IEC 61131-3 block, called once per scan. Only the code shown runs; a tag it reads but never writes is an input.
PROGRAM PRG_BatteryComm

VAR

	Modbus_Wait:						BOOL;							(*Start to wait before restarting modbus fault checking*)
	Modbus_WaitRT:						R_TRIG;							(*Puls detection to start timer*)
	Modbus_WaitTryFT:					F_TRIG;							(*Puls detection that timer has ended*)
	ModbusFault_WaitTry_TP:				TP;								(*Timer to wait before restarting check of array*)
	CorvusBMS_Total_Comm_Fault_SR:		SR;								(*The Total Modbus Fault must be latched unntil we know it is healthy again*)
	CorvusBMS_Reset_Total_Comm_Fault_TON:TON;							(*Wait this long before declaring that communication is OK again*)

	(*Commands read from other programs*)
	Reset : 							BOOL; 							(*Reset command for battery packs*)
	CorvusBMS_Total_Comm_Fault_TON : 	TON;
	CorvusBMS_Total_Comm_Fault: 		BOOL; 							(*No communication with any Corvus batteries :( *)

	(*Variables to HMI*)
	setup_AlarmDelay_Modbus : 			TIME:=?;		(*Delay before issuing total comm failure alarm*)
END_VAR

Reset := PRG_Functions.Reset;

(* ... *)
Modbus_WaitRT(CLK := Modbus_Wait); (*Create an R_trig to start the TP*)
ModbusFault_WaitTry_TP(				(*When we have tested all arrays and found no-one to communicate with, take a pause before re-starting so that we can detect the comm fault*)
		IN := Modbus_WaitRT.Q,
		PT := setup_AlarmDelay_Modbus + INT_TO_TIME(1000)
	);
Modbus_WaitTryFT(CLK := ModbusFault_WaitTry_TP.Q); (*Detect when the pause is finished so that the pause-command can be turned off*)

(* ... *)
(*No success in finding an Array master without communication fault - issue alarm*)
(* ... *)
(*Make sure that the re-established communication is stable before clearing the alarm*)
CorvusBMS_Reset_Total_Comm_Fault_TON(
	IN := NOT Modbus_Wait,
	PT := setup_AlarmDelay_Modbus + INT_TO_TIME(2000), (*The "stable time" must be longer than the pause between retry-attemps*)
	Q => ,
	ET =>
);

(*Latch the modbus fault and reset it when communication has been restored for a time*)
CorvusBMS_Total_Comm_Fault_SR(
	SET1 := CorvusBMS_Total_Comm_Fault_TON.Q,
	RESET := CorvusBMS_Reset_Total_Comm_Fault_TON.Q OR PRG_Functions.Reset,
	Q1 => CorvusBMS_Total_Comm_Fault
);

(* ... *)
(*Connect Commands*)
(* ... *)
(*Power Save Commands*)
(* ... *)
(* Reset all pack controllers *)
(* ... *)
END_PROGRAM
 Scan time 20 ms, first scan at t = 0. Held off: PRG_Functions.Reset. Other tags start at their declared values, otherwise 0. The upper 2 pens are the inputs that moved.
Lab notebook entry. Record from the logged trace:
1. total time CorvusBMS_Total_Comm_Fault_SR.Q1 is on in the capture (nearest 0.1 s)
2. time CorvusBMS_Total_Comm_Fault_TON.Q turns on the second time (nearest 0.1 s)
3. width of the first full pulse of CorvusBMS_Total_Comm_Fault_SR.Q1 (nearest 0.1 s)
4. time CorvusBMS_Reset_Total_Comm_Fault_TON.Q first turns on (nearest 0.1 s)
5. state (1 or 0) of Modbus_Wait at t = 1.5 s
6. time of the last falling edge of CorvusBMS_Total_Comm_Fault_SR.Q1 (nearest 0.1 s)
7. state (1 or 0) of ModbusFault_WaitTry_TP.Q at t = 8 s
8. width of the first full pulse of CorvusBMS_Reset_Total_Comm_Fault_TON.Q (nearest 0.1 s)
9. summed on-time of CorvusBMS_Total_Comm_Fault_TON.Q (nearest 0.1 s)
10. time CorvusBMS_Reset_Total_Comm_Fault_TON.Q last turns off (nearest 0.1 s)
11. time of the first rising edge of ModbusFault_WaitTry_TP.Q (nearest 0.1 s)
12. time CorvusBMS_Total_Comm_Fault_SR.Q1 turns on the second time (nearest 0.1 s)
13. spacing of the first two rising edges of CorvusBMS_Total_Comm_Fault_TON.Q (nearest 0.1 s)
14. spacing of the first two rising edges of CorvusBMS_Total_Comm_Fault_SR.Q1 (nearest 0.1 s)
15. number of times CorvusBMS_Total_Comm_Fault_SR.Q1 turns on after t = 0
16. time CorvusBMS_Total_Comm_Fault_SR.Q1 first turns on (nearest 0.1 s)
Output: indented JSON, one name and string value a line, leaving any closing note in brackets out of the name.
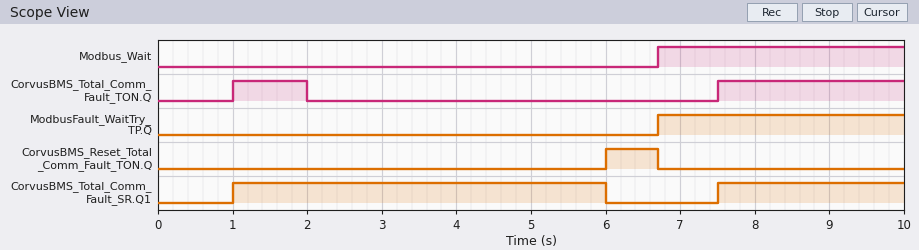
{
  "total time CorvusBMS_Total_Comm_Fault_SR.Q1 is on in the capture": "7.5 s",
  "time CorvusBMS_Total_Comm_Fault_TON.Q turns on the second time": "7.5 s",
  "width of the first full pulse of CorvusBMS_Total_Comm_Fault_SR.Q1": "5.0 s",
  "time CorvusBMS_Reset_Total_Comm_Fault_TON.Q first turns on": "6.0 s",
  "state (1 or 0) of Modbus_Wait at t = 1.5 s": "0",
  "time of the last falling edge of CorvusBMS_Total_Comm_Fault_SR.Q1": "6.0 s",
  "state (1 or 0) of ModbusFault_WaitTry_TP.Q at t = 8 s": "1",
  "width of the first full pulse of CorvusBMS_Reset_Total_Comm_Fault_TON.Q": "0.7 s",
  "summed on-time of CorvusBMS_Total_Comm_Fault_TON.Q": "3.5 s",
  "time CorvusBMS_Reset_Total_Comm_Fault_TON.Q last turns off": "6.7 s",
  "time of the first rising edge of ModbusFault_WaitTry_TP.Q": "6.7 s",
  "time CorvusBMS_Total_Comm_Fault_SR.Q1 turns on the second time": "7.5 s",
  "spacing of the first two rising edges of CorvusBMS_Total_Comm_Fault_TON.Q": "6.5 s",
  "spacing of the first two rising edges of CorvusBMS_Total_Comm_Fault_SR.Q1": "6.5 s",
  "number of times CorvusBMS_Total_Comm_Fault_SR.Q1 turns on after t = 0": "2",
  "time CorvusBMS_Total_Comm_Fault_SR.Q1 first turns on": "1.0 s"
}
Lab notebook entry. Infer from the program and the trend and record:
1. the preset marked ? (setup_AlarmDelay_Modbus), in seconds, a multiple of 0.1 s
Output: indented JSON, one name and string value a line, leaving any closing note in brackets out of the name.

{
  "the preset marked ? (setup_AlarmDelay_Modbus), in seconds, a multiple of 0.1 s": "4.0 s"
}
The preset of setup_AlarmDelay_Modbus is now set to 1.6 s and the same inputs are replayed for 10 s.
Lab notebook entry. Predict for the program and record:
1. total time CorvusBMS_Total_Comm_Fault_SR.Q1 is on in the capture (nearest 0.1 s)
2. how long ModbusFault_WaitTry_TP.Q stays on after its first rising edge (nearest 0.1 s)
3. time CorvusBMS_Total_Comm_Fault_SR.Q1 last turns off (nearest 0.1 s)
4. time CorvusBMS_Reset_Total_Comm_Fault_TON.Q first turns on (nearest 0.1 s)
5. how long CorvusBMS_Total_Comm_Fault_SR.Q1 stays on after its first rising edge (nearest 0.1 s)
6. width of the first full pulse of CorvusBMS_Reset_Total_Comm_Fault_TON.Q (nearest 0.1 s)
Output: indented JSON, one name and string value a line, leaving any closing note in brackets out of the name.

{
  "total time CorvusBMS_Total_Comm_Fault_SR.Q1 is on in the capture": "5.1 s",
  "how long ModbusFault_WaitTry_TP.Q stays on after its first rising edge": "2.6 s",
  "time CorvusBMS_Total_Comm_Fault_SR.Q1 last turns off": "3.6 s",
  "time CorvusBMS_Reset_Total_Comm_Fault_TON.Q first turns on": "3.6 s",
  "how long CorvusBMS_Total_Comm_Fault_SR.Q1 stays on after its first rising edge": "2.6 s",
  "width of the first full pulse of CorvusBMS_Reset_Total_Comm_Fault_TON.Q": "3.1 s"
}
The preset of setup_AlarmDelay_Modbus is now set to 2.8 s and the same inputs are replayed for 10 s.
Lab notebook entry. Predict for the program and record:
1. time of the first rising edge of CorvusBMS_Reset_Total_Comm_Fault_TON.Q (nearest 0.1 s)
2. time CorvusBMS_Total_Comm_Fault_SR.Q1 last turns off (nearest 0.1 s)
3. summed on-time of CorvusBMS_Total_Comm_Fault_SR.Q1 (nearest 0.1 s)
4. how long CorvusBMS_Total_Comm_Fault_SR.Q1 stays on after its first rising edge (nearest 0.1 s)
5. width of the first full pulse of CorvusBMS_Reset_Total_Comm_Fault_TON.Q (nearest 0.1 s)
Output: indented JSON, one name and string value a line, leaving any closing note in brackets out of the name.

{
  "time of the first rising edge of CorvusBMS_Reset_Total_Comm_Fault_TON.Q": "4.8 s",
  "time CorvusBMS_Total_Comm_Fault_SR.Q1 last turns off": "4.8 s",
  "summed on-time of CorvusBMS_Total_Comm_Fault_SR.Q1": "6.3 s",
  "how long CorvusBMS_Total_Comm_Fault_SR.Q1 stays on after its first rising edge": "3.8 s",
  "width of the first full pulse of CorvusBMS_Reset_Total_Comm_Fault_TON.Q": "1.9 s"
}
